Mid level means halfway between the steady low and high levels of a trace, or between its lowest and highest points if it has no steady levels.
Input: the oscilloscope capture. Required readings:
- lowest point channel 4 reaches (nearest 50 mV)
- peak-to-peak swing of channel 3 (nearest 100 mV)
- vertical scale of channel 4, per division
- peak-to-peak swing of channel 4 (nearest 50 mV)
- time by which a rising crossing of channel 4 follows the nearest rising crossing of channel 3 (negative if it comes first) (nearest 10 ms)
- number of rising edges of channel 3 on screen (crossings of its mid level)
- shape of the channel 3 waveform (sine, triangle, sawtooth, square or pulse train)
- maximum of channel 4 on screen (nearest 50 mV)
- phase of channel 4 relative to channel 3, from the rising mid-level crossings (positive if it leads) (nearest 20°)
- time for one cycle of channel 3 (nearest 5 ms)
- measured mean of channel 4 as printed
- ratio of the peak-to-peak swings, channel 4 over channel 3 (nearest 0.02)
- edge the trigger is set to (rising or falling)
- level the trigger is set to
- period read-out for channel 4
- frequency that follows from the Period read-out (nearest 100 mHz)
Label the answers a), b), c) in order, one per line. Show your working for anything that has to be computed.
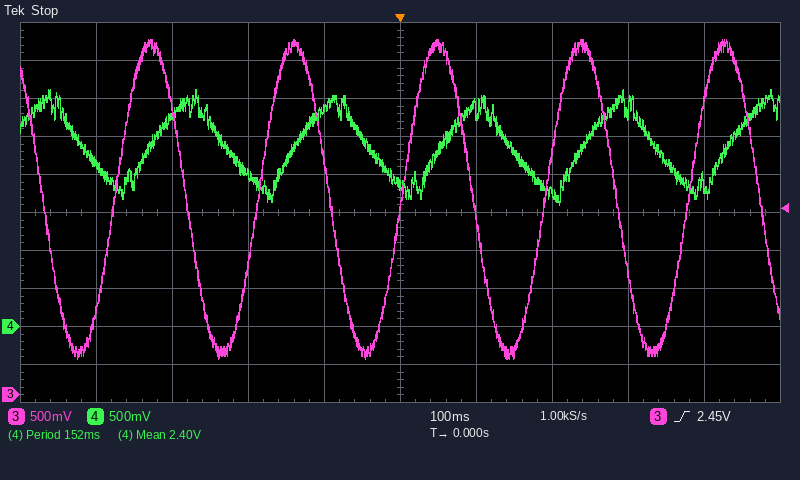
a) 1.60 V
b) 4.20 V
c) 500 mV
d) 3.10 V − (1.60 V) = 1.50 V
e) +50 ms
f) 5
g) sine
h) 3.10 V
i) −360° × (+50 ms) / 190 ms ≈ -94.7°, so -100° to the nearest 20°
j) 190 ms
k) 2.40 V
l) 1.50 V / 4.20 V ≈ 0.36
m) rising
n) 2.45 V
o) 152 ms
p) 1 / 152 ms ≈ 6.6 Hz
